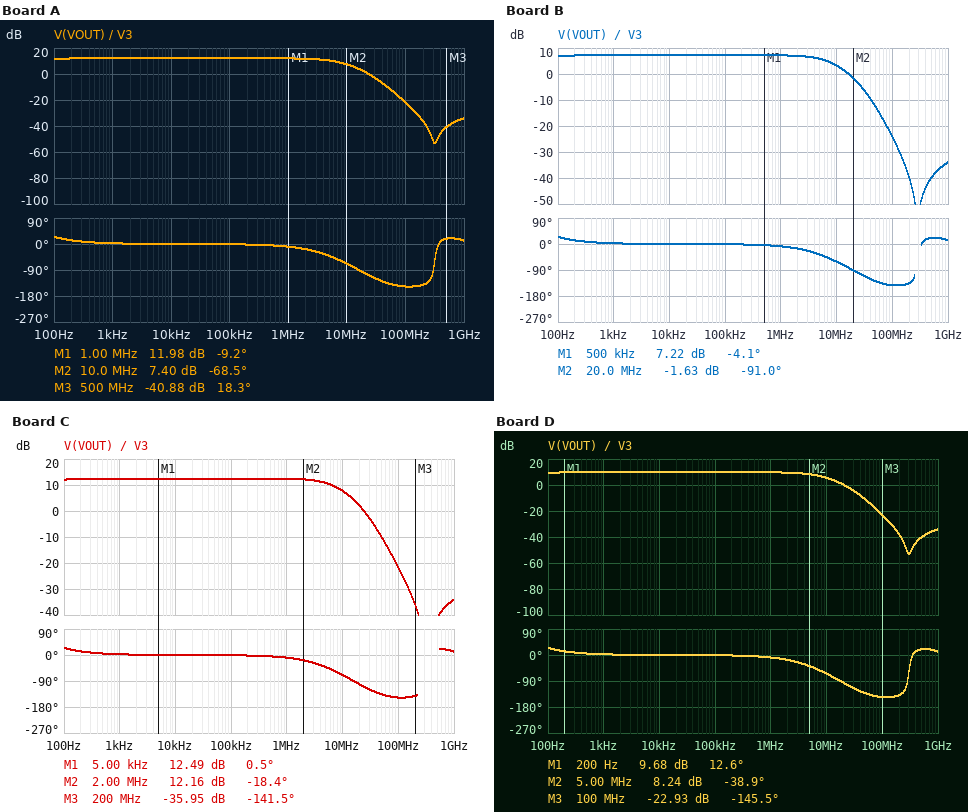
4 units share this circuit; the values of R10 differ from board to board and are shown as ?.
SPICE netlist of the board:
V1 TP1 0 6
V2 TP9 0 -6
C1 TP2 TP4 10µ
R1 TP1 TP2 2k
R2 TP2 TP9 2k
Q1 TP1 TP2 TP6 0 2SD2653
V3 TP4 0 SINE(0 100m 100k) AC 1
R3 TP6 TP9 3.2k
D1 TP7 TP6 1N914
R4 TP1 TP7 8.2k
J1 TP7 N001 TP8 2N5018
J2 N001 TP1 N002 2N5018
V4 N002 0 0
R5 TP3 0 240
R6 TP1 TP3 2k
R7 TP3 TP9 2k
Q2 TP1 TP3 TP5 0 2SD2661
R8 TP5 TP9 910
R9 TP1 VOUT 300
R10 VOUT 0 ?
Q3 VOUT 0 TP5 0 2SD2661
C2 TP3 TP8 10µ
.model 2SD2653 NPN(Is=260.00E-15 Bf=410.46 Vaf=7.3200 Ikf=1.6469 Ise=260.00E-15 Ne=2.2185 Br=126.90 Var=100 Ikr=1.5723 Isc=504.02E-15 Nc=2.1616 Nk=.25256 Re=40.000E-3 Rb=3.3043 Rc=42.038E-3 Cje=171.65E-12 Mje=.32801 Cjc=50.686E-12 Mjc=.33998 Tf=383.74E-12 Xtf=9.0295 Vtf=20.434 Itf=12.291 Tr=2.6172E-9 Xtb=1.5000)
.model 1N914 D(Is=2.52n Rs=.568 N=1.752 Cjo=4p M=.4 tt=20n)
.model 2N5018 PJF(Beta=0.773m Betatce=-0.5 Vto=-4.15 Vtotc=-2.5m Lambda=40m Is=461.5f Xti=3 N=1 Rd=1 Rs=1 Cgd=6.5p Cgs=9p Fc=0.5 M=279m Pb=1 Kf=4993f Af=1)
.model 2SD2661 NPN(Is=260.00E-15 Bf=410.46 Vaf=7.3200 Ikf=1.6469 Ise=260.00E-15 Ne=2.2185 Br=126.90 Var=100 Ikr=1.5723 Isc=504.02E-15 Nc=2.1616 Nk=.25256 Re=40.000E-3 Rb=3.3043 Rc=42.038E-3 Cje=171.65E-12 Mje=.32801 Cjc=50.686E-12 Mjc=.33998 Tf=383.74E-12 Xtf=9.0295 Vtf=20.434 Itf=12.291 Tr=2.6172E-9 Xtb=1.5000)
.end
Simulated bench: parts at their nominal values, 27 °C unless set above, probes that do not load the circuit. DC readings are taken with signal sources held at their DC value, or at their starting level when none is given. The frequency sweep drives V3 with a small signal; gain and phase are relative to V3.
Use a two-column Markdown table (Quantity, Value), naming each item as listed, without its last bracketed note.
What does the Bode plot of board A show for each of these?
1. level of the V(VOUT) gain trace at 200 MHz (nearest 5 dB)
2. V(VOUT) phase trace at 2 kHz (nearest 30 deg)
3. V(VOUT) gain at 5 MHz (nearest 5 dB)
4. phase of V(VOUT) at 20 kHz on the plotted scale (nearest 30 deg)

| Quantity | Value |
|---|---|
| level of the V(VOUT) gain trace at 200 MHz | -35 dB |
| V(VOUT) phase trace at 2 kHz | 0 deg |
| V(VOUT) gain at 5 MHz | 10 dB |
| phase of V(VOUT) at 20 kHz on the plotted scale | 0 deg |
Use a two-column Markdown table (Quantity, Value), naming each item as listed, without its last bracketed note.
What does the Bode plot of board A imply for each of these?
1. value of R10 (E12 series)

| Quantity | Value |
|---|---|
| value of R10 | 820 Ω |
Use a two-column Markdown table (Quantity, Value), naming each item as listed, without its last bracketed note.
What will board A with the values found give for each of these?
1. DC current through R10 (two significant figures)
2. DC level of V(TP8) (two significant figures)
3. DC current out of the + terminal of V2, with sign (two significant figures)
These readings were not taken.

| Quantity | Value |
|---|---|
| DC current through R10 | 4.6 mA |
| DC level of V(TP8) | 14 mV |
| DC current out of the + terminal of V2, with sign | -14 mA |
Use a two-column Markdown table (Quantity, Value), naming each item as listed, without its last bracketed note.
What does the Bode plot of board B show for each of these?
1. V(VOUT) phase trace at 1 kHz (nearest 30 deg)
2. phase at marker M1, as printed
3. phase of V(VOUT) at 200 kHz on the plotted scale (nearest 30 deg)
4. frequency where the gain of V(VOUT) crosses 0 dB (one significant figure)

| Quantity | Value |
|---|---|
| V(VOUT) phase trace at 1 kHz | 0 deg |
| phase at marker M1, as printed | -4.1 deg |
| phase of V(VOUT) at 200 kHz on the plotted scale | 0 deg |
| frequency where the gain of V(VOUT) crosses 0 dB | 20 MHz |
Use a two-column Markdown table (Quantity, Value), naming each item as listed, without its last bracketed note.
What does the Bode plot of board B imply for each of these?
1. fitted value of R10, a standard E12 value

| Quantity | Value |
|---|---|
| fitted value of R10, a standard E12 value | 220 Ω |
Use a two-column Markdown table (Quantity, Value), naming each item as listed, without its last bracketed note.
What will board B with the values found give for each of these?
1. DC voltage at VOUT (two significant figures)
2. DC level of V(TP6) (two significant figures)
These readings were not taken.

| Quantity | Value |
|---|---|
| DC voltage at VOUT | 2.2 V |
| DC level of V(TP6) | -560 mV |
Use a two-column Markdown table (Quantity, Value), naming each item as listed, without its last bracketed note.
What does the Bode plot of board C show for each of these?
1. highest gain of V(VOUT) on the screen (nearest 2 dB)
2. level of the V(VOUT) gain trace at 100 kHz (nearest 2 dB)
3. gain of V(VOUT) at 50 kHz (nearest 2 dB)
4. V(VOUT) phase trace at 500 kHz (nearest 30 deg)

| Quantity | Value |
|---|---|
| highest gain of V(VOUT) on the screen | 12 dB |
| level of the V(VOUT) gain trace at 100 kHz | 12 dB |
| gain of V(VOUT) at 50 kHz | 12 dB |
| V(VOUT) phase trace at 500 kHz | 0 deg |
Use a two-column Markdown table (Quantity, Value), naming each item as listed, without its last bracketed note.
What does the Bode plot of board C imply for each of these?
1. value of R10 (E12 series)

| Quantity | Value |
|---|---|
| value of R10 | 1 kΩ |
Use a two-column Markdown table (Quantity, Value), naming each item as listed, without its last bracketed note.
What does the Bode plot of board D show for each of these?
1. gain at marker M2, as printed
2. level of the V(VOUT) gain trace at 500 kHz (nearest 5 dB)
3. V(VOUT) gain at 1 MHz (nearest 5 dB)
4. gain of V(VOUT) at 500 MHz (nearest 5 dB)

| Quantity | Value |
|---|---|
| gain at marker M2, as printed | 8.24 dB |
| level of the V(VOUT) gain trace at 500 kHz | 10 dB |
| V(VOUT) gain at 1 MHz | 10 dB |
| gain of V(VOUT) at 500 MHz | -40 dB |
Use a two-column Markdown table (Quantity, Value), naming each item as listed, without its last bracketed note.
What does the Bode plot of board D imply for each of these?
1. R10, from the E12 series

| Quantity | Value |
|---|---|
| R10, from the E12 series | 390 Ω |
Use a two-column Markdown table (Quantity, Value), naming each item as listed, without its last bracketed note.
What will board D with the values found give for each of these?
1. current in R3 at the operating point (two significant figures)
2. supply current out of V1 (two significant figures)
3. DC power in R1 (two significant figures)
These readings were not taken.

| Quantity | Value |
|---|---|
| current in R3 at the operating point | 1.7 mA |
| supply current out of V1 | 21 mA |
| DC power in R1 | 18 mW |
